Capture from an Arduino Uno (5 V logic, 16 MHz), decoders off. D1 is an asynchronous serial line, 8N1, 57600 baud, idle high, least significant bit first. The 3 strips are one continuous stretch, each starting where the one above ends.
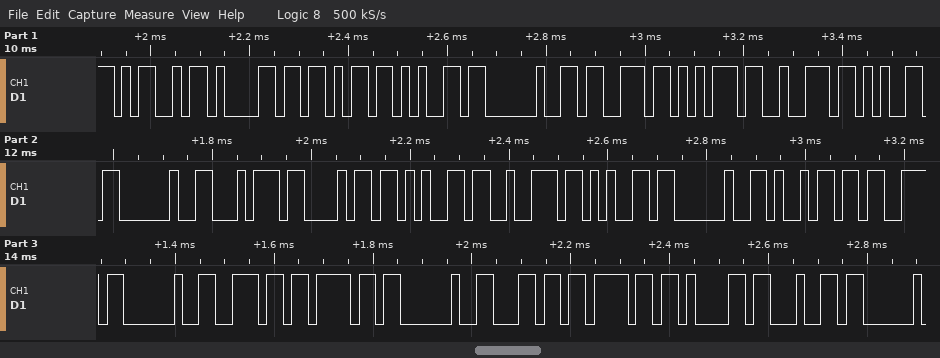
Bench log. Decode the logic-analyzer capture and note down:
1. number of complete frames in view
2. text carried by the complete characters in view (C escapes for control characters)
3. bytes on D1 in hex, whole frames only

26
"Make sure there is no load"
0x4D 0x61 0x6B 0x65 0x20 0x73 0x75 0x72 0x65 0x20 0x74 0x68 0x65 0x72 0x65 0x20 0x69 0x73 0x20 0x6E 0x6F 0x20 0x6C 0x6F 0x61 0x64
